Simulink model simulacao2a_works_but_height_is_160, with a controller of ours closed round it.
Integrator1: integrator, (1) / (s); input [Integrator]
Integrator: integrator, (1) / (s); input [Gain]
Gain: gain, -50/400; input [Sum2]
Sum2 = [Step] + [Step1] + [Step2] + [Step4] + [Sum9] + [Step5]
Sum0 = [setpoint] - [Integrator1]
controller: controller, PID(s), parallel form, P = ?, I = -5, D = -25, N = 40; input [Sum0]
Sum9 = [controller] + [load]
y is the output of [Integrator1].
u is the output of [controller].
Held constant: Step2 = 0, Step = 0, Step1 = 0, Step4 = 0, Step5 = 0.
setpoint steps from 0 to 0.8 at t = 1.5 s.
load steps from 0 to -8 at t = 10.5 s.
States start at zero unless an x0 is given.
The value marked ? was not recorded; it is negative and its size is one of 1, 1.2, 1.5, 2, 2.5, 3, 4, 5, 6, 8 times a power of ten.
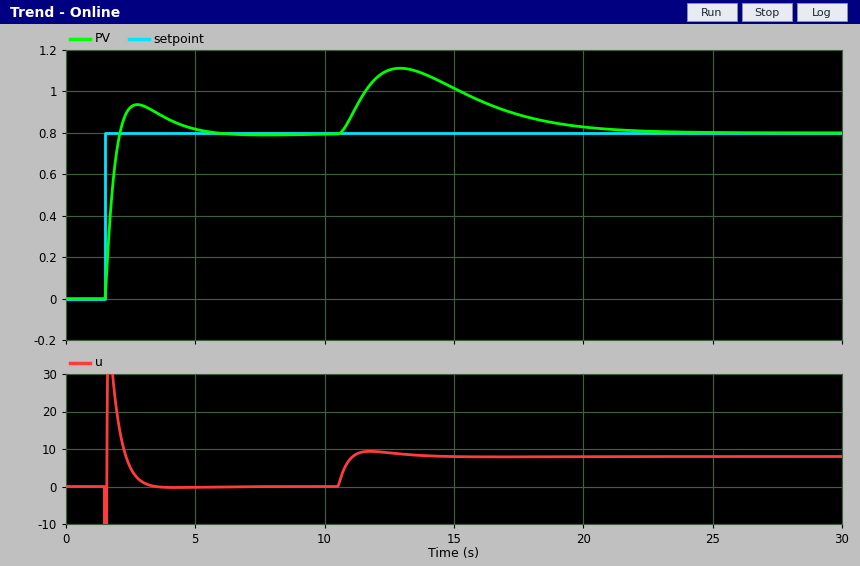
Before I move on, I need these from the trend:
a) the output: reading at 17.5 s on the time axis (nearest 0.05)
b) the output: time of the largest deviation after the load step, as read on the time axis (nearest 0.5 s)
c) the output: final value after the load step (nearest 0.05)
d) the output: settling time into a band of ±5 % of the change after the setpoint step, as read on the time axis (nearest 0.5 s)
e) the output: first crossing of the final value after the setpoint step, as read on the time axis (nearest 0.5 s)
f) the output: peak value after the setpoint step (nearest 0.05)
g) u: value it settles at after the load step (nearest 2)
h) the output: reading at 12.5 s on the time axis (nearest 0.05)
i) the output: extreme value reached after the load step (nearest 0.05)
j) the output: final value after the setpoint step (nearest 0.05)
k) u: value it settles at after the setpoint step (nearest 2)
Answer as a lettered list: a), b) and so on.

a) 0.90
b) 13.0 s
c) 0.80
d) 4.5 s
e) 2.0 s
f) 0.95
g) 8
h) 1.10
i) 1.10
j) 0.80
k) 0
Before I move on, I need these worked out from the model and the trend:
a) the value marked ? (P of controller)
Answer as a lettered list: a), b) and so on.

a) -20
